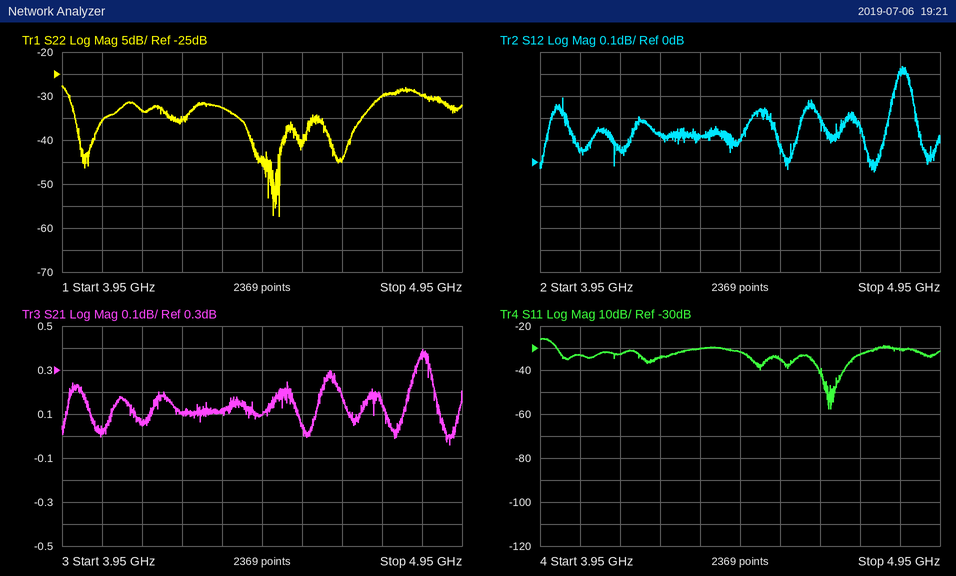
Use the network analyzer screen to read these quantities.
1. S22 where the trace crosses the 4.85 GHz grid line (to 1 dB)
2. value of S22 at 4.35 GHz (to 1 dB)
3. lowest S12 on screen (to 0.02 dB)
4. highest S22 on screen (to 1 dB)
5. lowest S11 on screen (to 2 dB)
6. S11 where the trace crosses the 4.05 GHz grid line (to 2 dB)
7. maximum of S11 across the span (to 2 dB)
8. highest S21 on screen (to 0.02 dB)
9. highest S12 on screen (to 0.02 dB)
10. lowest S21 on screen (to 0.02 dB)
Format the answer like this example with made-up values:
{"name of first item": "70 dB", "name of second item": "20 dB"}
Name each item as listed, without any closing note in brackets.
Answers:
{"S22 where the trace crosses the 4.85 GHz grid line": "-30 dB", "value of S22 at 4.35 GHz": "-33 dB", "lowest S12 on screen": "-0.04 dB", "highest S22 on screen": "-28 dB", "lowest S11 on screen": "-58 dB", "S11 where the trace crosses the 4.05 GHz grid line": "-34 dB", "maximum of S11 across the span": "-26 dB", "highest S21 on screen": "0.40 dB", "highest S12 on screen": "0.44 dB", "lowest S21 on screen": "-0.04 dB"}
